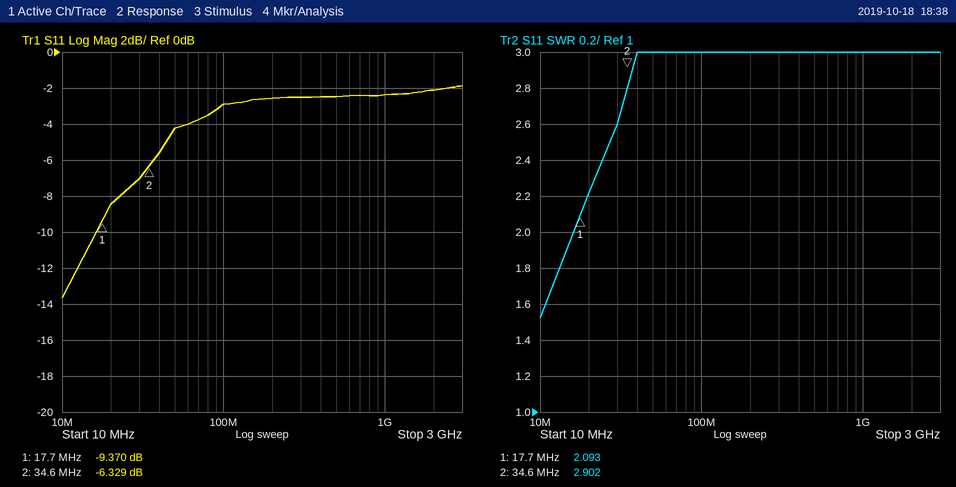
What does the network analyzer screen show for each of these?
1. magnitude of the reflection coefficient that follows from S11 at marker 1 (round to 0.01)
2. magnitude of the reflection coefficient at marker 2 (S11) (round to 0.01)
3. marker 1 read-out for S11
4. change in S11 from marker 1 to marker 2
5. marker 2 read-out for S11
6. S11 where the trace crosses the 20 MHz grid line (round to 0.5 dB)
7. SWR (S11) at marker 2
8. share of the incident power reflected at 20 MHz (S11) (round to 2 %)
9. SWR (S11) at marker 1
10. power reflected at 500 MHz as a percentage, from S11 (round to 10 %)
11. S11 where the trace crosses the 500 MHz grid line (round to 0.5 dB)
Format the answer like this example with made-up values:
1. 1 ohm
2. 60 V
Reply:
1. 0.34
2. 0.48
3. -9.370 dB
4. 3.041 dB
5. -6.329 dB
6. -8.5 dB
7. 2.902
8. 14 %
9. 2.093
10. 60 %
11. -2.5 dB
